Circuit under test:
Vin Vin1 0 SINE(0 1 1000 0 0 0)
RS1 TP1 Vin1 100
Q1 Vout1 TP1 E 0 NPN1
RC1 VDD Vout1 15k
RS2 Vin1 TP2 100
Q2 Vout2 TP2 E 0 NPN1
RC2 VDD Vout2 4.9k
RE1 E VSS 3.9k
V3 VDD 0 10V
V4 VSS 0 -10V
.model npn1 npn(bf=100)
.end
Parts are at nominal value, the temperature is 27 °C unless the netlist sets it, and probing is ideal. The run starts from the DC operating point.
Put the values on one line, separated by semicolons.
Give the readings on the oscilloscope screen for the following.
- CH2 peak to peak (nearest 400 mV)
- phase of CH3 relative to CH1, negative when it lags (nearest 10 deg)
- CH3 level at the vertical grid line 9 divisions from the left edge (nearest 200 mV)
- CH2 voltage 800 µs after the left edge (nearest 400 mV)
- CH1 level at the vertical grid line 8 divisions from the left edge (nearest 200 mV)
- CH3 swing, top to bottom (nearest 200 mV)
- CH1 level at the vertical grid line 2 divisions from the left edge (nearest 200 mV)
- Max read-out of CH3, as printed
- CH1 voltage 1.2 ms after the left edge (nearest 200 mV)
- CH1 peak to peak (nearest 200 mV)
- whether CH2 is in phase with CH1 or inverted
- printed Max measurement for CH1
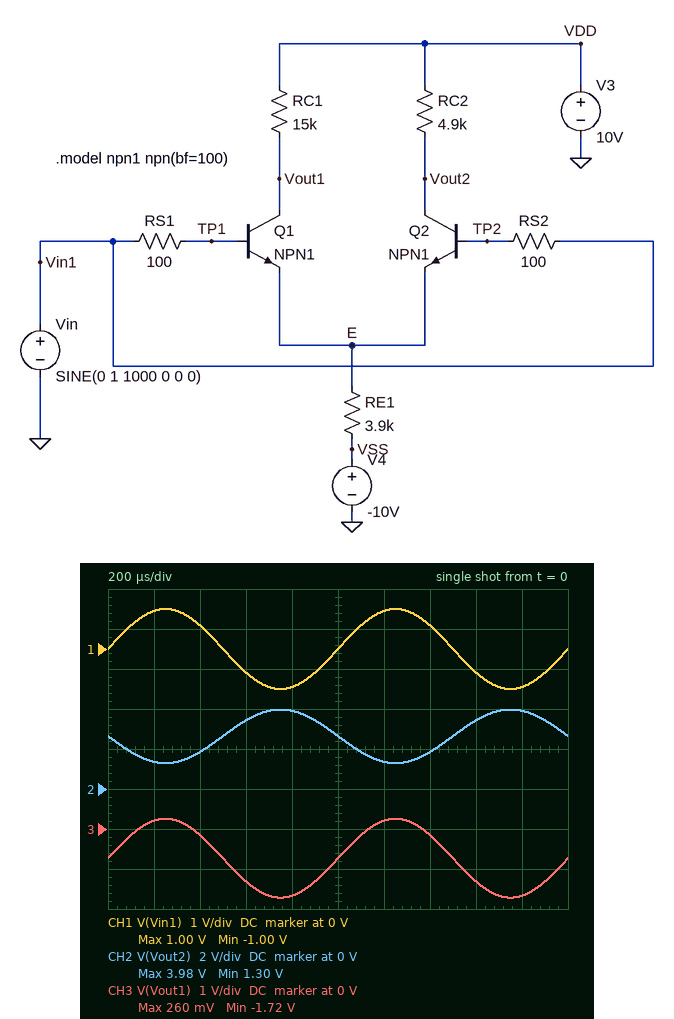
2.8 V; 0 deg; -1.6 V; 4.0 V; -600 mV; 2.0 V; 600 mV; 260 mV; 1.0 V; 2.0 V; inverted; 1.00 V
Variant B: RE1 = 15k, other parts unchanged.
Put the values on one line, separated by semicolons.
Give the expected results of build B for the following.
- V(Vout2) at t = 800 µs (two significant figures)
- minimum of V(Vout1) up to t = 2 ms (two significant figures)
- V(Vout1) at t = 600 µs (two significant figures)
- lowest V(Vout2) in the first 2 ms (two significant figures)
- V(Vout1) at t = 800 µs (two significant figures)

8.7 V; 4.9 V; 5.7 V; 8.3 V; 5.9 V
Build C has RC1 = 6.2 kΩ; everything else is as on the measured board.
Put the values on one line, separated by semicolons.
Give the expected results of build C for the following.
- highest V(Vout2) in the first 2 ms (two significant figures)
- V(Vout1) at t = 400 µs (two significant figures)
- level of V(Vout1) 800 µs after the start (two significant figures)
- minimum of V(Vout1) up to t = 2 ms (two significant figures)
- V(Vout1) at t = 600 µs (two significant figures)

4.9 V; 2.3 V; 3.5 V; 2.0 V; 3.2 V
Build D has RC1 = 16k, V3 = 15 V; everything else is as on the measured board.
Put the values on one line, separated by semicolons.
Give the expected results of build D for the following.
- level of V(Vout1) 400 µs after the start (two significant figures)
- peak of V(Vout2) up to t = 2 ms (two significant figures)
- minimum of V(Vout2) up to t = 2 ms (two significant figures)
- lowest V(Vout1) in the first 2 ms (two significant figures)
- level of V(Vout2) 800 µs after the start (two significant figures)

-130 mV; 9.9 V; 7.3 V; -1.6 V; 9.8 V
